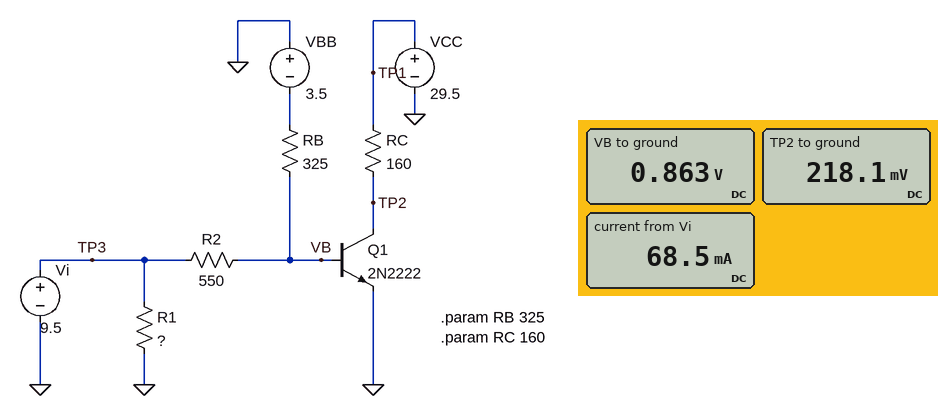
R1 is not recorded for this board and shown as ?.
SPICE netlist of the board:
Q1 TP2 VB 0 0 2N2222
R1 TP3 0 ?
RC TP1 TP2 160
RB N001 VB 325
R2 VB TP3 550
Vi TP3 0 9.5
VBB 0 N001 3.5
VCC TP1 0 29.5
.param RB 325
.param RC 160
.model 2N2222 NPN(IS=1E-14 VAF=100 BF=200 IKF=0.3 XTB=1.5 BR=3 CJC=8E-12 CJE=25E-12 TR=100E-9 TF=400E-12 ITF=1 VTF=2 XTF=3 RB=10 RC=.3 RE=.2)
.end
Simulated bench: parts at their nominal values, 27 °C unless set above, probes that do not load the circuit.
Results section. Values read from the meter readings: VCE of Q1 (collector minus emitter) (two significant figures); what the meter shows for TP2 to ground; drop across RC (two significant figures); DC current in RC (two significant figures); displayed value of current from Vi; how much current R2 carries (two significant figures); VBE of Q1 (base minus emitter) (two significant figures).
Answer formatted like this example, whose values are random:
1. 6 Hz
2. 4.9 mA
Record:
1. 220 mV
2. 218.1 mV
3. 29 V
4. 180 mA
5. 68.5 mA
6. 16 mA
7. 860 mV
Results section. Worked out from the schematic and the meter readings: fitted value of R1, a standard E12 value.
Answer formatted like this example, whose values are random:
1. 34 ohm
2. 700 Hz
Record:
1. 180 Ω
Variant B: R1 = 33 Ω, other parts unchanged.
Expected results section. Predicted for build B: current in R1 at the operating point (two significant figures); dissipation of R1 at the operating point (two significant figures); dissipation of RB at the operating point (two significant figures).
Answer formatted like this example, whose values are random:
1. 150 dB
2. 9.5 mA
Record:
1. 290 mA
2. 2.7 W
3. 59 mW
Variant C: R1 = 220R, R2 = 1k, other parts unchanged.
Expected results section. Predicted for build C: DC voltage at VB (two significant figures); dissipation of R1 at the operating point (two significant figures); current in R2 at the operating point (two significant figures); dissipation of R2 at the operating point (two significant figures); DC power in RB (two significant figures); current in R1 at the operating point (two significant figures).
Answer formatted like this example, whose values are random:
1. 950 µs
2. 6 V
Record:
1. -310 mV
2. 410 mW
3. 9.8 mA
4. 96 mW
5. 31 mW
6. 43 mA
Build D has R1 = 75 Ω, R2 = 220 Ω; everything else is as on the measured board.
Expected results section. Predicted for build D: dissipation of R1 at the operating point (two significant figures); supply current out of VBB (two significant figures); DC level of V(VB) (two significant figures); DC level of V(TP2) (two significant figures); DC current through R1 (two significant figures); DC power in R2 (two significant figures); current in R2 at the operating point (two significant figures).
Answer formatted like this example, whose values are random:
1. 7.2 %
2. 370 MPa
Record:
1. 1.2 W
2. 14 mA
3. 1.1 V
4. 150 mV
5. 130 mA
6. 320 mW
7. 38 mA
